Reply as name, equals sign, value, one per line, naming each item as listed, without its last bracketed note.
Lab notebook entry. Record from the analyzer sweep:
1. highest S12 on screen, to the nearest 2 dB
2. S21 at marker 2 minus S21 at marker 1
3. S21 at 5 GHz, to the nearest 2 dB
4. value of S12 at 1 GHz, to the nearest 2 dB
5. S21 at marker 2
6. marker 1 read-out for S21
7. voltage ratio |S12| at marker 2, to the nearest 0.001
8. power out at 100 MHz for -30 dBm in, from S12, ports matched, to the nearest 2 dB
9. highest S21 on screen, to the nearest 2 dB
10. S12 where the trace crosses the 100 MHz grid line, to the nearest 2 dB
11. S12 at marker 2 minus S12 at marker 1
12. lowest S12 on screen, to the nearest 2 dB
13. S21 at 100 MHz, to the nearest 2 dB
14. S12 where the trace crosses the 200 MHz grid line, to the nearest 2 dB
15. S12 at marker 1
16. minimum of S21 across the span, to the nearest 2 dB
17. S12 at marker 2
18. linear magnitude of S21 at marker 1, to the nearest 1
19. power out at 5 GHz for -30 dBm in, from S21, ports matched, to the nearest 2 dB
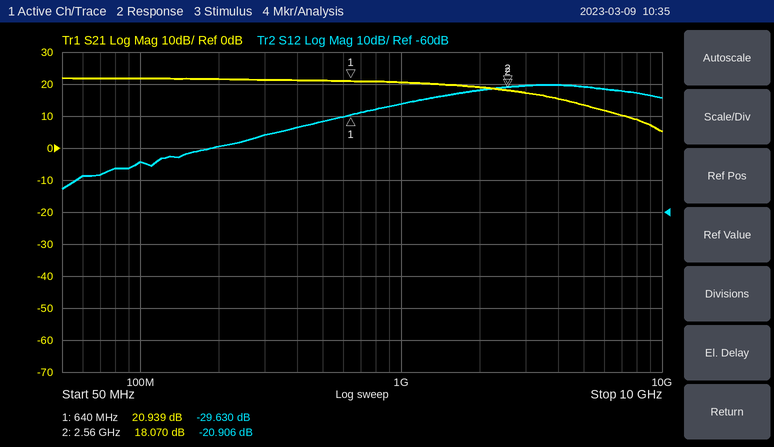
highest S12 on screen, to the nearest 2 dB = -20 dB
S21 at marker 2 minus S21 at marker 1 = -2.869 dB
S21 at 5 GHz, to the nearest 2 dB = 14 dB
value of S12 at 1 GHz, to the nearest 2 dB = -26 dB
S21 at marker 2 = 18.070 dB
marker 1 read-out for S21 = 20.939 dB
voltage ratio |S12| at marker 2, to the nearest 0.001 = 0.090
power out at 100 MHz for -30 dBm in, from S12, ports matched, to the nearest 2 dB = -74 dBm
highest S21 on screen, to the nearest 2 dB = 22 dB
S12 where the trace crosses the 100 MHz grid line, to the nearest 2 dB = -44 dB
S12 at marker 2 minus S12 at marker 1 = 8.724 dB
lowest S12 on screen, to the nearest 2 dB = -52 dB
S21 at 100 MHz, to the nearest 2 dB = 22 dB
S12 where the trace crosses the 200 MHz grid line, to the nearest 2 dB = -40 dB
S12 at marker 1 = -29.630 dB
minimum of S21 across the span, to the nearest 2 dB = 6 dB
S12 at marker 2 = -20.906 dB
linear magnitude of S21 at marker 1, to the nearest 1 = 11
power out at 5 GHz for -30 dBm in, from S21, ports matched, to the nearest 2 dB = -16 dBm
